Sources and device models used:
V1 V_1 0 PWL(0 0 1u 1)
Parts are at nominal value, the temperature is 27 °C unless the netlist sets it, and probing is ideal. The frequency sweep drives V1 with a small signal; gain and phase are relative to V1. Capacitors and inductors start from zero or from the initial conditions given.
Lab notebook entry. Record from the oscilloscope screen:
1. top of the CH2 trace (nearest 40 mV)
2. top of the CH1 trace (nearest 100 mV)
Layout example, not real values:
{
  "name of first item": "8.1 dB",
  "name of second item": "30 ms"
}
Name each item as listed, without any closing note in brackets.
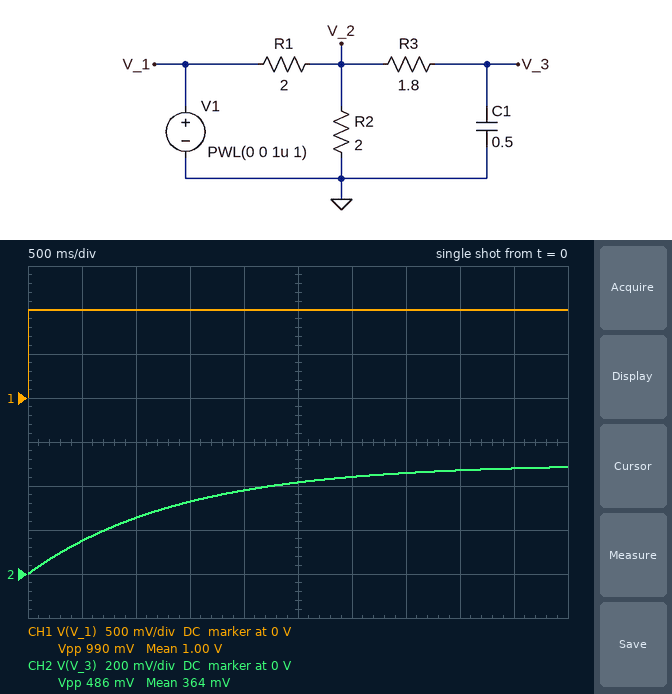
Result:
{
  "top of the CH2 trace": "480 mV",
  "top of the CH1 trace": "1.0 V"
}
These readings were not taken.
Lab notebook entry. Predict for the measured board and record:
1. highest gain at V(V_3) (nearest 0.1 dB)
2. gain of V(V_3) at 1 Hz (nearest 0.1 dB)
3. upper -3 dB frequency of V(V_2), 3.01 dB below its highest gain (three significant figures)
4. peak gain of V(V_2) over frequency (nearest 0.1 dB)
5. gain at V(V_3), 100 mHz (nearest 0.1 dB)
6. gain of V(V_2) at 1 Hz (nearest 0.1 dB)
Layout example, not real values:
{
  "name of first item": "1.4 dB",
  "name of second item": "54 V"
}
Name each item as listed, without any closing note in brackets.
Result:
{
  "highest gain at V(V_3)": "-6.0 dB",
  "gain of V(V_3) at 1 Hz": "-25.0 dB",
  "upper -3 dB frequency of V(V_2), 3.01 dB below its highest gain": "273 mHz",
  "peak gain of V(V_2) over frequency": "-6.0 dB",
  "gain at V(V_3), 100 mHz": "-8.5 dB",
  "gain of V(V_2) at 1 Hz": "-9.8 dB"
}
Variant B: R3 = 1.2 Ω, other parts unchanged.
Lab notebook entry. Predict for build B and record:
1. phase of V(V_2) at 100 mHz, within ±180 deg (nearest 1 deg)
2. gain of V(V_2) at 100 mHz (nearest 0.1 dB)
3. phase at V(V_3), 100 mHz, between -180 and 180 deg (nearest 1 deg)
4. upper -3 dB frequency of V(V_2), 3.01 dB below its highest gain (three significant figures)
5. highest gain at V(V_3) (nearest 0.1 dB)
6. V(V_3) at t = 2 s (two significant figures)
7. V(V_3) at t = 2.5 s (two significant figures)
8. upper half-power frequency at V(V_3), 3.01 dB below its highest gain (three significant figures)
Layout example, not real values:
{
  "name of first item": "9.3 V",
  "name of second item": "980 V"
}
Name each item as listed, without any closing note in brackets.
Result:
{
  "phase of V(V_2) at 100 mHz, within ±180 deg": "-14 deg",
  "gain of V(V_2) at 100 mHz": "-7.1 dB",
  "phase at V(V_3), 100 mHz, between -180 and 180 deg": "-35 deg",
  "upper -3 dB frequency of V(V_2), 3.01 dB below its highest gain": "227 mHz",
  "highest gain at V(V_3)": "-6.0 dB",
  "V(V_3) at t = 2 s": "420 mV",
  "V(V_3) at t = 2.5 s": "450 mV",
  "upper half-power frequency at V(V_3), 3.01 dB below its highest gain": "145 mHz"
}
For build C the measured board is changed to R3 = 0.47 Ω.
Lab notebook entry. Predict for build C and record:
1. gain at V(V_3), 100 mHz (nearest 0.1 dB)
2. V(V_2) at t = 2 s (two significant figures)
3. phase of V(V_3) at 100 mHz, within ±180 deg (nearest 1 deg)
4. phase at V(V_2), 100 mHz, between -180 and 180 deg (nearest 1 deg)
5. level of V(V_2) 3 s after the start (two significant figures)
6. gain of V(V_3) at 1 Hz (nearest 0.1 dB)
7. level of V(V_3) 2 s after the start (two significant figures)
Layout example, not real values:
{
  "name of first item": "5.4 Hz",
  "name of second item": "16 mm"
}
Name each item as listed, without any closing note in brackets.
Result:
{
  "gain at V(V_3), 100 mHz": "-6.9 dB",
  "V(V_2) at t = 2 s": "480 mV",
  "phase of V(V_3) at 100 mHz, within ±180 deg": "-25 deg",
  "phase at V(V_2), 100 mHz, between -180 and 180 deg": "-16 deg",
  "level of V(V_2) 3 s after the start": "490 mV",
  "gain of V(V_3) at 1 Hz": "-19.5 dB",
  "level of V(V_3) 2 s after the start": "470 mV"
}
